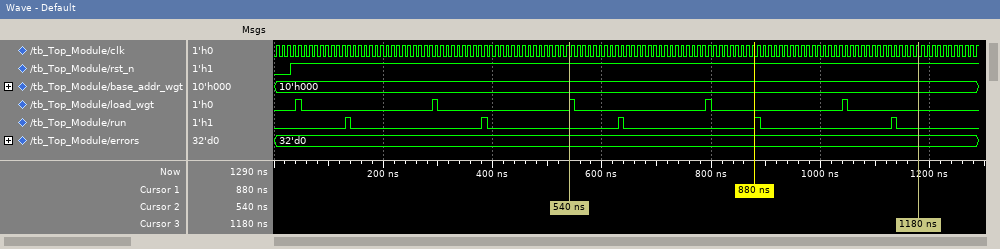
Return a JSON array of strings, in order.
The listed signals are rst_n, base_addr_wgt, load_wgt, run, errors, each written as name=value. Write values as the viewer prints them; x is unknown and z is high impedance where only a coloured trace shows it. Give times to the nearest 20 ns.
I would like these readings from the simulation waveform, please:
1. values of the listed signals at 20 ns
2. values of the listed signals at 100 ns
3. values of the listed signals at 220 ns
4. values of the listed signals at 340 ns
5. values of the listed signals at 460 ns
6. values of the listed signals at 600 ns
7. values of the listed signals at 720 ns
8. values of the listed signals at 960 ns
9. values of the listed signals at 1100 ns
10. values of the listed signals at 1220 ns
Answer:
["rst_n=0, base_addr_wgt=10'h000, load_wgt=0, run=0, errors=32'd0", "rst_n=1, base_addr_wgt=10'h000, load_wgt=0, run=0, errors=32'd0", "rst_n=1, base_addr_wgt=10'h000, load_wgt=0, run=0, errors=32'd0", "rst_n=1, base_addr_wgt=10'h000, load_wgt=0, run=0, errors=32'd0", "rst_n=1, base_addr_wgt=10'h000, load_wgt=0, run=0, errors=32'd0", "rst_n=1, base_addr_wgt=10'h000, load_wgt=0, run=0, errors=32'd0", "rst_n=1, base_addr_wgt=10'h000, load_wgt=0, run=0, errors=32'd0", "rst_n=1, base_addr_wgt=10'h000, load_wgt=0, run=0, errors=32'd0", "rst_n=1, base_addr_wgt=10'h000, load_wgt=0, run=0, errors=32'd0", "rst_n=1, base_addr_wgt=10'h000, load_wgt=0, run=0, errors=32'd0"]
